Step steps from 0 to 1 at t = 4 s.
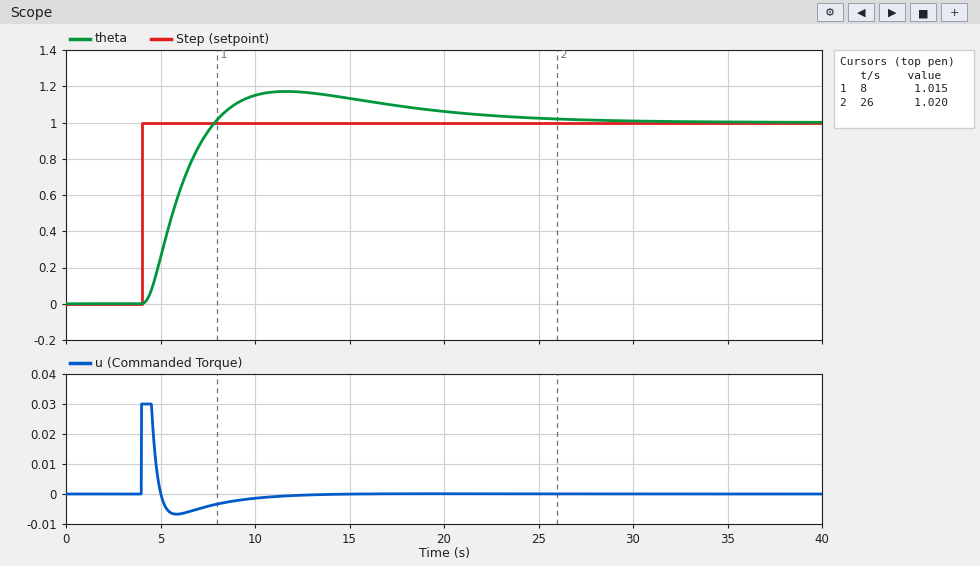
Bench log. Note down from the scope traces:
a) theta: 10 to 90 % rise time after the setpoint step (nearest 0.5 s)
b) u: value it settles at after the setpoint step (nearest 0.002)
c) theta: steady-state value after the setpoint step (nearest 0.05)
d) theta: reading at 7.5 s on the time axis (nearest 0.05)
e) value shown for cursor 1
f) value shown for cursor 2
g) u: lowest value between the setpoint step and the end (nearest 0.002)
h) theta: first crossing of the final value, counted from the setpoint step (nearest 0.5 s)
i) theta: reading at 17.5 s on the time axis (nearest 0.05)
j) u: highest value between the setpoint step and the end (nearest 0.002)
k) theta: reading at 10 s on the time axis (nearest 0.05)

2.5 s
0.000
1.00
0.95
1.015
1.020
-0.006
4.0 s
1.10
0.030
1.15
